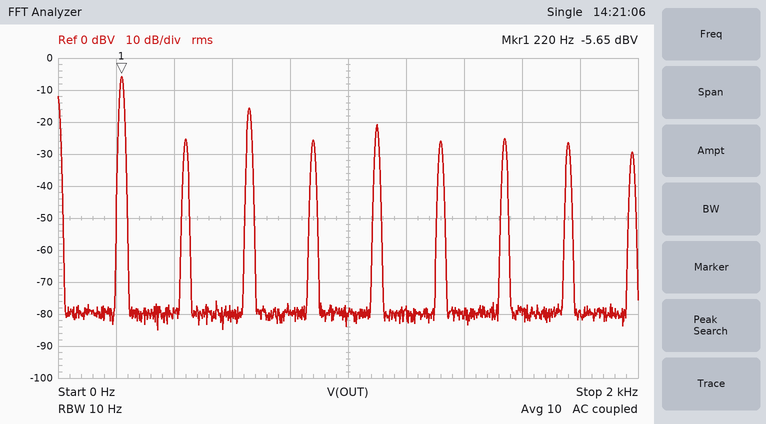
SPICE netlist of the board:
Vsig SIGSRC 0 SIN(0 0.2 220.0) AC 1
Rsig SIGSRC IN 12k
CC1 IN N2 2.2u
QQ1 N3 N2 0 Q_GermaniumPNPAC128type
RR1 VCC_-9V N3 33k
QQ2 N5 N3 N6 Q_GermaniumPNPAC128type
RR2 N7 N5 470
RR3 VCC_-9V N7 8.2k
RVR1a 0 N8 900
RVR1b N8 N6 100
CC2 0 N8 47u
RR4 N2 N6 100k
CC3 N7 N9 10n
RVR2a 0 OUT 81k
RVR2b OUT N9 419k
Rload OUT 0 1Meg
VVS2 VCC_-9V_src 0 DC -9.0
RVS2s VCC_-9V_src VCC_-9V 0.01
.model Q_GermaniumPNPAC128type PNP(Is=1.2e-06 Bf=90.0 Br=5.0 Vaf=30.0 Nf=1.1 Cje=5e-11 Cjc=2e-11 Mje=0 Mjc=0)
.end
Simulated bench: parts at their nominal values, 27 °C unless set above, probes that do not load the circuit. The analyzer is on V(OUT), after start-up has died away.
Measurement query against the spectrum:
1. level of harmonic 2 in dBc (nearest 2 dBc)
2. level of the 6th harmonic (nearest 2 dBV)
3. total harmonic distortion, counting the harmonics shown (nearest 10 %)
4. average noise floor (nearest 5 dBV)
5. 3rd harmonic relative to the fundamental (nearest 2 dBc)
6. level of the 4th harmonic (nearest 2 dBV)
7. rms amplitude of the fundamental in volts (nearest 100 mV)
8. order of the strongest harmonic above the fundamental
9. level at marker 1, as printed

-20 dBc
-26 dBV
40 %
-80 dBV
-10 dBc
-26 dBV
500 mV
3
-5.65 dBV
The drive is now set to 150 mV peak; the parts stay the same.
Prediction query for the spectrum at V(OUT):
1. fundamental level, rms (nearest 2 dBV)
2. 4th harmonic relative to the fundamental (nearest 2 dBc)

-6 dBV
-30 dBc
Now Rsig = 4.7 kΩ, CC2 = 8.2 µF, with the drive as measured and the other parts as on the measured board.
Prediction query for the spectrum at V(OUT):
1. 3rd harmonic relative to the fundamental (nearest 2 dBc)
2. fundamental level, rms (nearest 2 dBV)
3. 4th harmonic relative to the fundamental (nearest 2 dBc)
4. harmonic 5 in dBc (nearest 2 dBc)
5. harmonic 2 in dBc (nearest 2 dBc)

-16 dBc
-6 dBV
-12 dBc
-24 dBc
-8 dBc
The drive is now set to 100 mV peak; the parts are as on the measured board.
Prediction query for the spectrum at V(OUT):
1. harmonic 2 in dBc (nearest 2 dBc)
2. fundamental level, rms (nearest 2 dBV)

-26 dBc
-6 dBV
